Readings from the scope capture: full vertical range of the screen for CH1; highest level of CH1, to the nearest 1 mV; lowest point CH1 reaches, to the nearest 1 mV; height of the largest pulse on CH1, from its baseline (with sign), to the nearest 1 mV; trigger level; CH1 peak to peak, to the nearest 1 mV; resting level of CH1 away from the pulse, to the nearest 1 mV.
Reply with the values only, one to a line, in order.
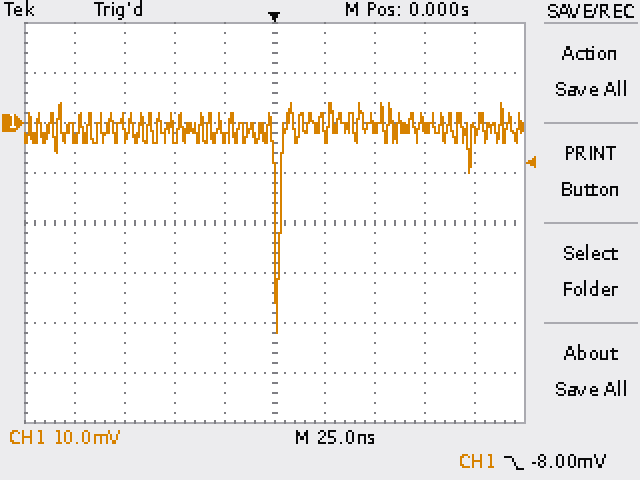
80 mV
4 mV
-42 mV
-41 mV
-8.00 mV
46 mV
-1 mV
